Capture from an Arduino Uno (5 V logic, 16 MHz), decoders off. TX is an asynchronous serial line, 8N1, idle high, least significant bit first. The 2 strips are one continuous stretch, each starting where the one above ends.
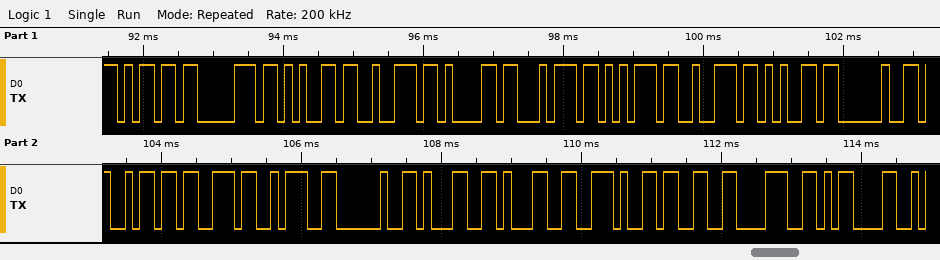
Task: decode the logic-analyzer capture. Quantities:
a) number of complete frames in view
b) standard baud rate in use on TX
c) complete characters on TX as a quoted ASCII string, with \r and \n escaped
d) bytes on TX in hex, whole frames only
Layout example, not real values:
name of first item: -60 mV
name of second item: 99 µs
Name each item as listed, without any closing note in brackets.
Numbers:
number of complete frames in view: 20
standard baud rate in use on TX: 9600 baud
complete characters on TX as a quoted ASCII string, with \r and \n escaped: "mperature is: 11.38\r"
bytes on TX in hex, whole frames only: 6D 70 65 72 61 74 75 72 65 20 69 73 3A 20 31 31 2E 33 38 0D
